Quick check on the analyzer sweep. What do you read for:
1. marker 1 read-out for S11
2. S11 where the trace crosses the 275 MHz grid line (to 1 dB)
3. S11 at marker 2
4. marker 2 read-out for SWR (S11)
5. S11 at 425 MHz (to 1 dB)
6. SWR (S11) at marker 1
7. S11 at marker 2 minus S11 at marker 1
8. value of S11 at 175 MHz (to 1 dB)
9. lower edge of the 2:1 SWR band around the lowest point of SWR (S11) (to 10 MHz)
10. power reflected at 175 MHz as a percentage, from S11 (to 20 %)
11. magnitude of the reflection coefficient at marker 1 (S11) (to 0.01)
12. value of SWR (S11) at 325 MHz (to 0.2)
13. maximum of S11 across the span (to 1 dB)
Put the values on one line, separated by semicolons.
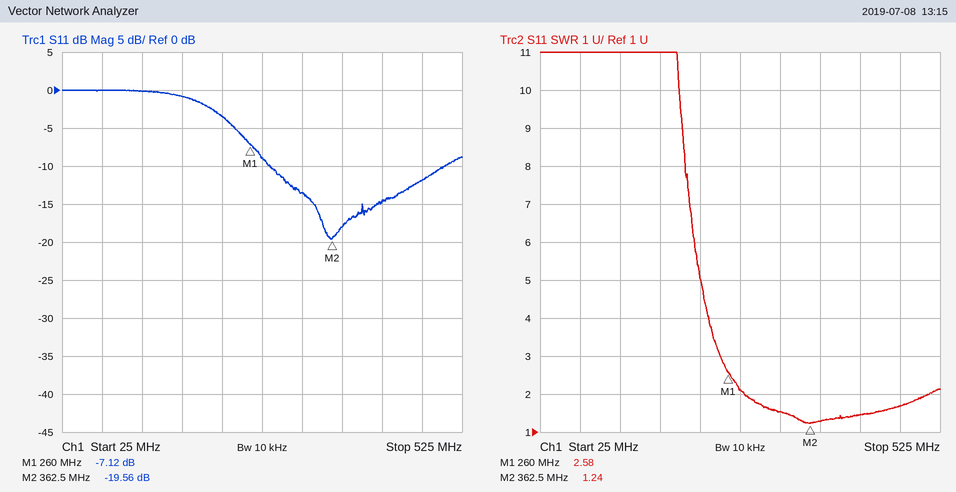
-7.12 dB; -9 dB; -19.56 dB; 1.24; -15 dB; 2.58; -12.44 dB; -1 dB; 280 MHz; 80 %; 0.44; 1.6; 0 dB
